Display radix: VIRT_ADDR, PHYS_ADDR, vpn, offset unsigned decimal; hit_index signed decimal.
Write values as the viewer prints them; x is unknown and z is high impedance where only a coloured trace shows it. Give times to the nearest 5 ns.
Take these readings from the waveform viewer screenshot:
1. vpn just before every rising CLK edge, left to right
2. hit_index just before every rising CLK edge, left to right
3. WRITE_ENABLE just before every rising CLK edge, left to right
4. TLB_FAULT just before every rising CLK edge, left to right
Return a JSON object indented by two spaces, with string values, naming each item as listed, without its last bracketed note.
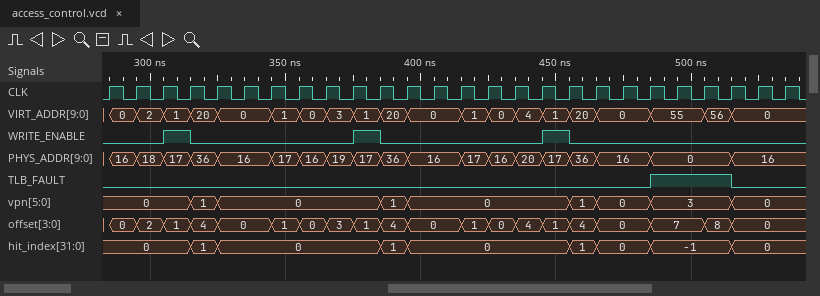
{
  "vpn just before every rising CLK edge, left to right": "0, 0, 0, 0, 1, 0, 0, 0, 0, 0, 0, 1, 0, 0, 0, 0, 0, 0, 1, 0, 0, 3, 3, 3, 0, 0",
  "hit_index just before every rising CLK edge, left to right": "0, 0, 0, 0, 1, 0, 0, 0, 0, 0, 0, 1, 0, 0, 0, 0, 0, 0, 1, 0, 0, -1, -1, -1, 0, 0",
  "WRITE_ENABLE just before every rising CLK edge, left to right": "0 0 0 1 0 0 0 0 0 0 1 0 0 0 0 0 0 1 0 0 0 0 0 0 0 0",
  "TLB_FAULT just before every rising CLK edge, left to right": "0 0 0 0 0 0 0 0 0 0 0 0 0 0 0 0 0 0 0 0 0 1 1 1 0 0"
}
